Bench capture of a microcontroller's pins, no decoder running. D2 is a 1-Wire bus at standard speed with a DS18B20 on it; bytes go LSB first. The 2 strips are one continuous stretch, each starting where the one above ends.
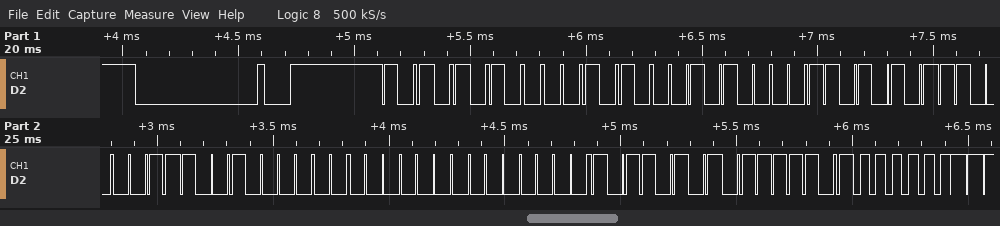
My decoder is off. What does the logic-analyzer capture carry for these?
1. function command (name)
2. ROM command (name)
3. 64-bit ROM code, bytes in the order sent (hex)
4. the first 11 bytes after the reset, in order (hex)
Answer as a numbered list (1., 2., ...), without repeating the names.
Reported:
1. Read Scratchpad
2. Match ROM
3. 28 0A AB C3 09 00 00 AD
4. 55 28 0A AB C3 09 00 00 AD BE C0
